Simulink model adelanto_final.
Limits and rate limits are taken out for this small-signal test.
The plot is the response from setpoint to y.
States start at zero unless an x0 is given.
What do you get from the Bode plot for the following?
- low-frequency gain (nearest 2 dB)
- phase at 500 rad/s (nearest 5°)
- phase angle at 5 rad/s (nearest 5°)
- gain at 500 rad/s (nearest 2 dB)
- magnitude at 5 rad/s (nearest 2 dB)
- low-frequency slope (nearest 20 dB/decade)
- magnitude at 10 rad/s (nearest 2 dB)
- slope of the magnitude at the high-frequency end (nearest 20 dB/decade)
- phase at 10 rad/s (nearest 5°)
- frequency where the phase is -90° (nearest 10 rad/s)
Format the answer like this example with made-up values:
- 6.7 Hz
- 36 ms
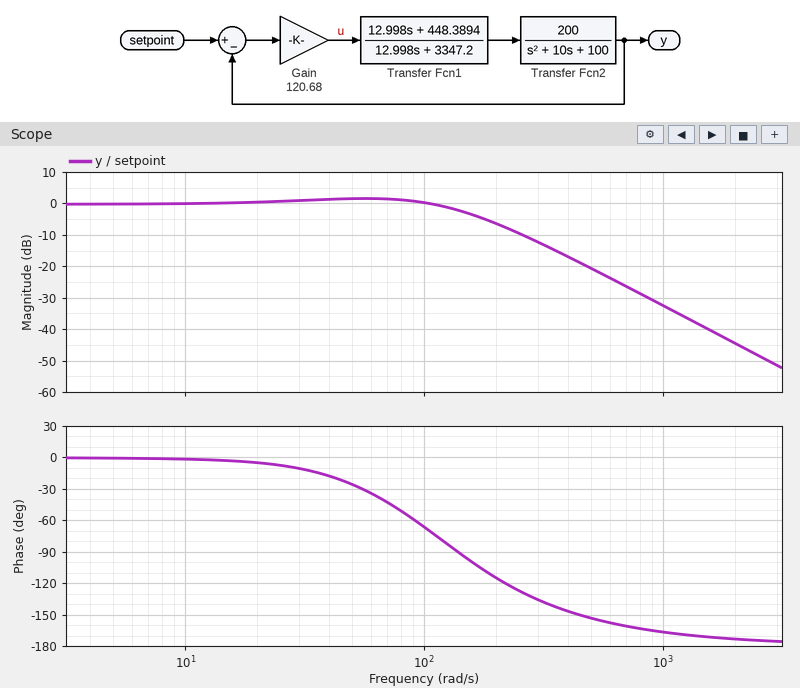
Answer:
- 0 dB
- -155°
- 0°
- -20 dB
- 0 dB
- 0 dB/decade
- 0 dB
- -40 dB/decade
- 0°
- 140 rad/s
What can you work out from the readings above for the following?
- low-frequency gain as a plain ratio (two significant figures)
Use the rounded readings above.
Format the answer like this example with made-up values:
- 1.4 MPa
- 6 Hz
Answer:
- 1.0
